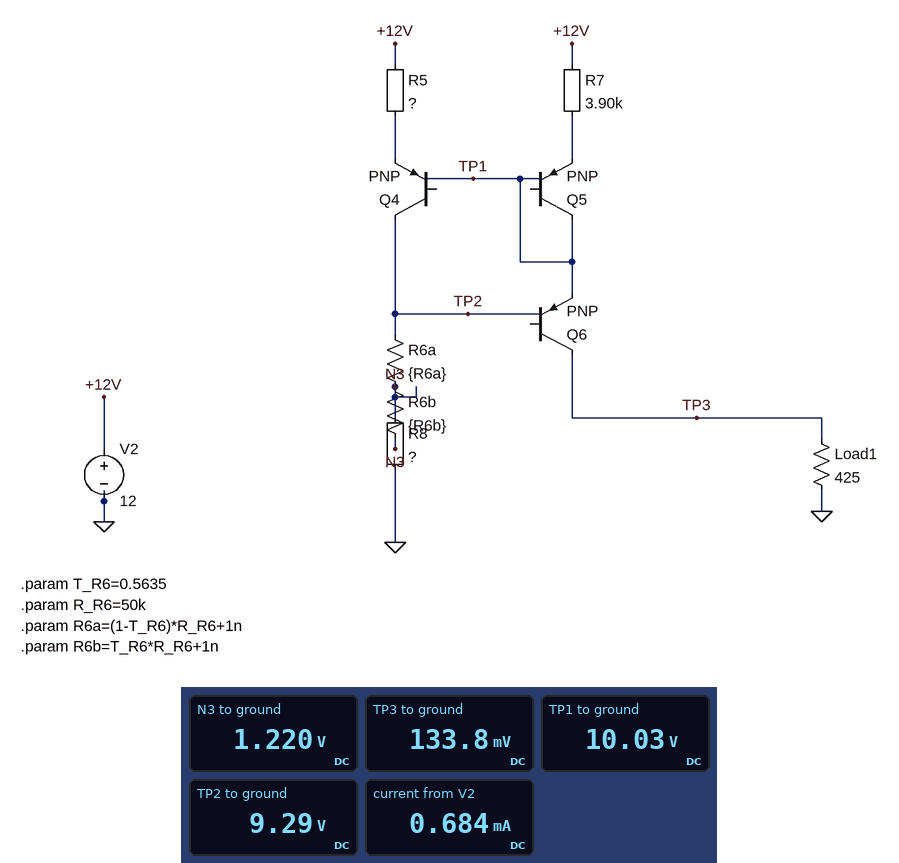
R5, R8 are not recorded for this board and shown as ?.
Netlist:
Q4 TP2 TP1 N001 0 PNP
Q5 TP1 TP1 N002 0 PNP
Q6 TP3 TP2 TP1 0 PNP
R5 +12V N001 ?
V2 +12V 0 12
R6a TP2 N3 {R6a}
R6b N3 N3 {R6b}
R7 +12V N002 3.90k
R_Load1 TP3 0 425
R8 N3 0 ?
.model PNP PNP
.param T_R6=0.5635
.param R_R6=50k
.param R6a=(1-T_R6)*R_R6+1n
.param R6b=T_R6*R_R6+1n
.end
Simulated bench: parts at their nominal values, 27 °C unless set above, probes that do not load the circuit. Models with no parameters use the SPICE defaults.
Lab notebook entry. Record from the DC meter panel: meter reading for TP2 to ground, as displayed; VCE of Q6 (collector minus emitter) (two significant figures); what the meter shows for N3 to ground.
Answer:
9.29 V
-9.9 V
1.220 V
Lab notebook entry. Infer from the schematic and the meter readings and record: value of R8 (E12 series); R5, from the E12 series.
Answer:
3.3 kΩ
3.3 kΩ
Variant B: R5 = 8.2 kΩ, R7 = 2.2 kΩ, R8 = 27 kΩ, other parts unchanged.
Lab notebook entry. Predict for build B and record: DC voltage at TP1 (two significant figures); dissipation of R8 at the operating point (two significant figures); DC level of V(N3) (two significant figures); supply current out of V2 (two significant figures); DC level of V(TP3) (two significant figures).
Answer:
9.8 V
920 µW
5.0 V
840 µA
280 mV
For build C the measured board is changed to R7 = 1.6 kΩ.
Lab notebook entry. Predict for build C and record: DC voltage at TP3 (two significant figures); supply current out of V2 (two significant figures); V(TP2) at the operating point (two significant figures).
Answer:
310 mV
1.1 mA
9.3 V
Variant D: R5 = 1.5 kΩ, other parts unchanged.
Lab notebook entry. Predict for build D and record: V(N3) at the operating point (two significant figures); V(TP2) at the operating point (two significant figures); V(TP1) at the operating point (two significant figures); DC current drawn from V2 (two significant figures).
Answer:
1.3 V
9.9 V
11 V
560 µA
